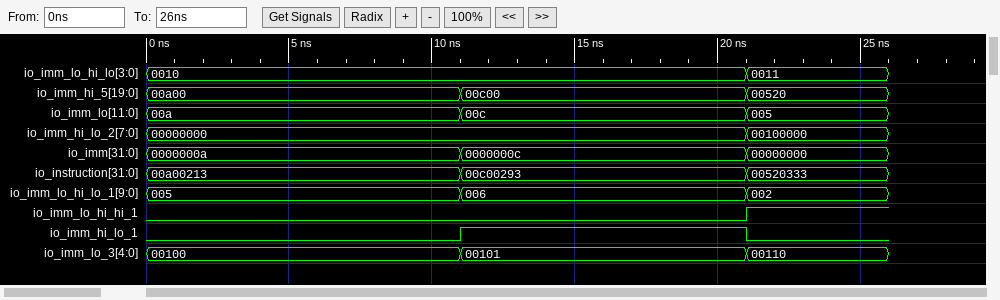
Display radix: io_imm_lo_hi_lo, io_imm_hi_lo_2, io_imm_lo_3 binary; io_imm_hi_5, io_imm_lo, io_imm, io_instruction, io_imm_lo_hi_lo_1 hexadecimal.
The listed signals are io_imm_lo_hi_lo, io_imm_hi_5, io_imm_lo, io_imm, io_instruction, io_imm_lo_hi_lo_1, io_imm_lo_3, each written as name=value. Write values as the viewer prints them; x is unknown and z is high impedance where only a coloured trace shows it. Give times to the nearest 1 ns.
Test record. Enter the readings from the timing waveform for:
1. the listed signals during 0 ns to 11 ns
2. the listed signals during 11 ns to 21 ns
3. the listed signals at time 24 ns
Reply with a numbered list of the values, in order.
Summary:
1. io_imm_lo_hi_lo=0010, io_imm_hi_5=00a00, io_imm_lo=00a, io_imm=0000000a, io_instruction=00a00213, io_imm_lo_hi_lo_1=005, io_imm_lo_3=00100
2. io_imm_lo_hi_lo=0010, io_imm_hi_5=00c00, io_imm_lo=00c, io_imm=0000000c, io_instruction=00c00293, io_imm_lo_hi_lo_1=006, io_imm_lo_3=00101
3. io_imm_lo_hi_lo=0011, io_imm_hi_5=00520, io_imm_lo=005, io_imm=00000000, io_instruction=00520333, io_imm_lo_hi_lo_1=002, io_imm_lo_3=00110
